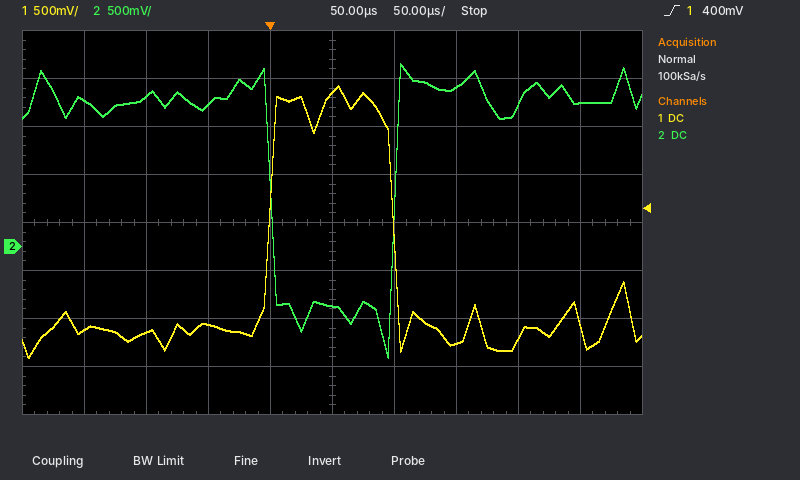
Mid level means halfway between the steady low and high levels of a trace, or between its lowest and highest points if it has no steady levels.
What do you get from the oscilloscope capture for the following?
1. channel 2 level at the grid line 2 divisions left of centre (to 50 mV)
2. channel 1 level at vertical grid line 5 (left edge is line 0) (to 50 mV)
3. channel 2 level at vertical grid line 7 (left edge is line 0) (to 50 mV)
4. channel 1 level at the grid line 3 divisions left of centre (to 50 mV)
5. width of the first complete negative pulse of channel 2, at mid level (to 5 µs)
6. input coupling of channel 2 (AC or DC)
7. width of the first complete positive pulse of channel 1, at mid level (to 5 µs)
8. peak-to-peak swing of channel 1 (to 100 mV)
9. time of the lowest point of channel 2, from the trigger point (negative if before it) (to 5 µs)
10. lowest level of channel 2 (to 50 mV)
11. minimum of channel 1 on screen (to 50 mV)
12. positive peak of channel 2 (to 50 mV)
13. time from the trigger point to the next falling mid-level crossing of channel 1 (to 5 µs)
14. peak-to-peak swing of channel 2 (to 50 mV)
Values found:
1.50 V
1.60 V
1.65 V
-900 mV
100 µs
DC
100 µs
2.80 V
+95 µs
-1.15 V
-1.15 V
1.90 V
100 µs
3.05 V
